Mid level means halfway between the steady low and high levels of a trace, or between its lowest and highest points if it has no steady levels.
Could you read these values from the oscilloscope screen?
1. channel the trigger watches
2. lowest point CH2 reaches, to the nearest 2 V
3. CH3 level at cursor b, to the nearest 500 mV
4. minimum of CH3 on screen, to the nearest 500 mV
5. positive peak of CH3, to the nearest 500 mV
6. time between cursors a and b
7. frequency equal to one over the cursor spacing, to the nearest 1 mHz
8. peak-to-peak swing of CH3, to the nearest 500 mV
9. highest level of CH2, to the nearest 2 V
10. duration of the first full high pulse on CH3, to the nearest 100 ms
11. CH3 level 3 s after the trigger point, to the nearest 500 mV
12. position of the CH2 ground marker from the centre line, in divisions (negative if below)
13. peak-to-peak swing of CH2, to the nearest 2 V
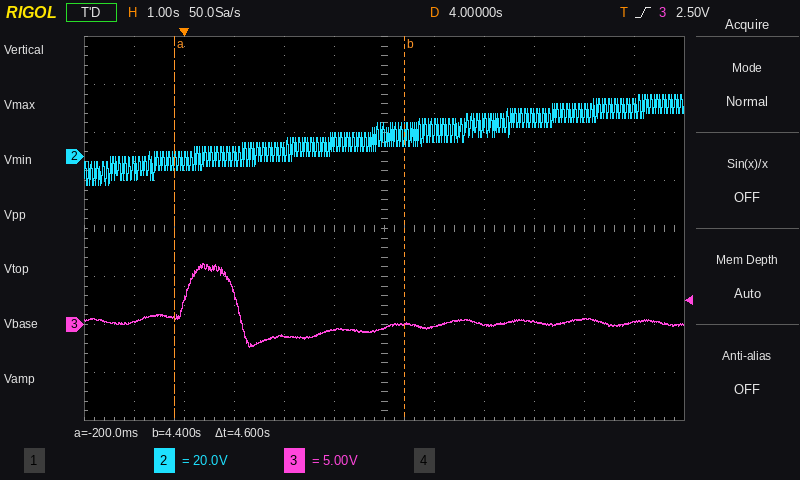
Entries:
CH3
-12 V
0.0 V
-2.5 V
6.5 V
4.6 s
217 mHz
9.0 V
26 V
1.1 s
-500 mV
+1.5 div
38 V
